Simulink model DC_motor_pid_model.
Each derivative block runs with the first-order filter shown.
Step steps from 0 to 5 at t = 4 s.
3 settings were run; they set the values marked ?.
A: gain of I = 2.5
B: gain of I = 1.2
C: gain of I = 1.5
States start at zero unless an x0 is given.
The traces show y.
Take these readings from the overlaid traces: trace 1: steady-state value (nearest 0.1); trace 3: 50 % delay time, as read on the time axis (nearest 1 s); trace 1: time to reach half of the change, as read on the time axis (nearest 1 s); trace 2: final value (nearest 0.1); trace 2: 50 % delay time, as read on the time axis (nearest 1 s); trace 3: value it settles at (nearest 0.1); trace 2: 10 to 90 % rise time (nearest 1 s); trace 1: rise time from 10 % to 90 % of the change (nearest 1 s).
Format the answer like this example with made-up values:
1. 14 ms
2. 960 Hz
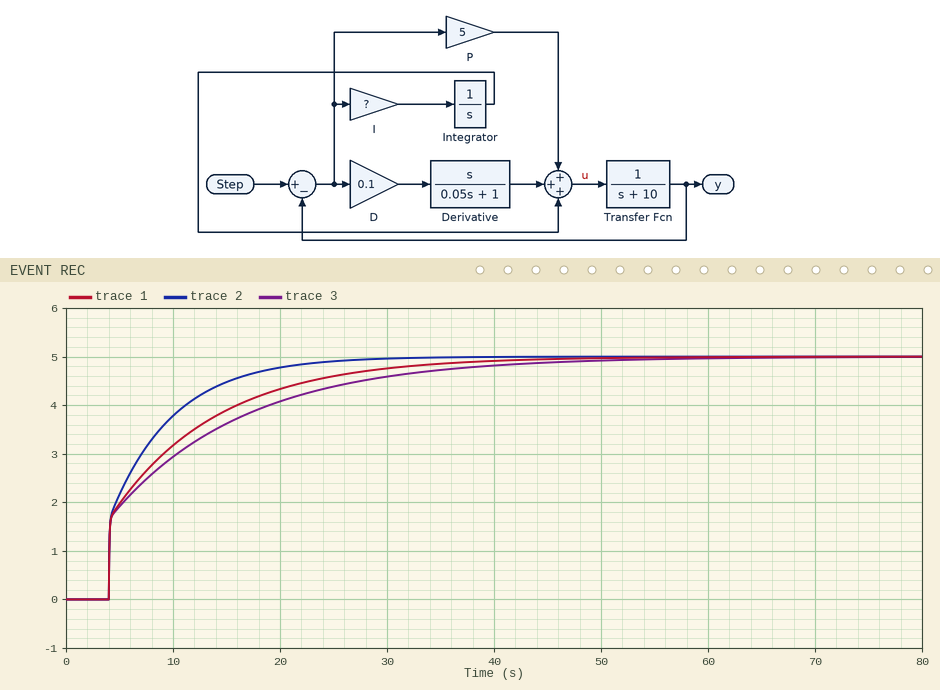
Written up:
1. 5.0
2. 8 s
3. 7 s
4. 5.0
5. 6 s
6. 5.0
7. 11 s
8. 19 s
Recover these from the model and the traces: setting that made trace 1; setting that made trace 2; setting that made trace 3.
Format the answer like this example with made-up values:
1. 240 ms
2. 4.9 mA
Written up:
1. C
2. A
3. B
